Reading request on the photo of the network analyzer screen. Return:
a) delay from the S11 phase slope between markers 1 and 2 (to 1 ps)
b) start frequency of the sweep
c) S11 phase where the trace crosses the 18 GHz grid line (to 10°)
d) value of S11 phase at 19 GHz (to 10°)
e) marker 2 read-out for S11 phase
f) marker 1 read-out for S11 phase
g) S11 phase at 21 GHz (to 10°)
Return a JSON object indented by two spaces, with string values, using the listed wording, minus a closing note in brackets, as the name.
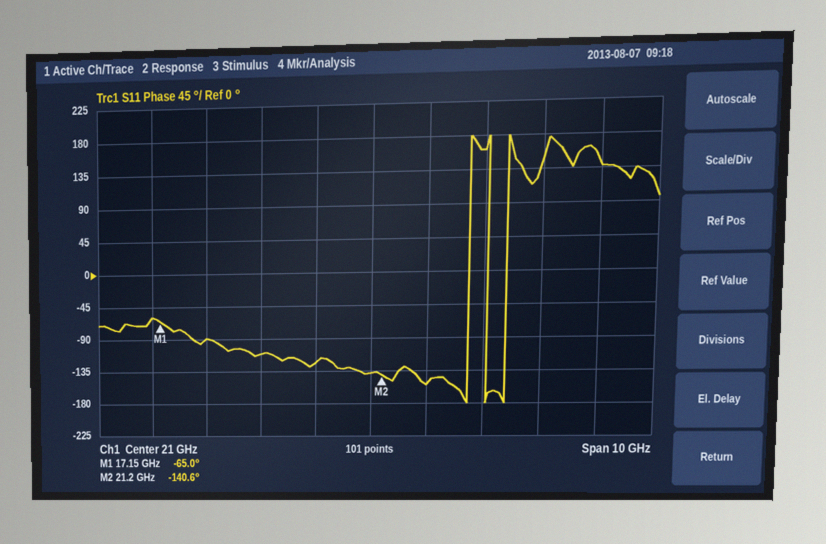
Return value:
{
  "delay from the S11 phase slope between markers 1 and 2": "52 ps",
  "start frequency of the sweep": "16 GHz",
  "S11 phase where the trace crosses the 18 GHz grid line": "-90°",
  "value of S11 phase at 19 GHz": "-110°",
  "marker 2 read-out for S11 phase": "-140.6°",
  "marker 1 read-out for S11 phase": "-65.0°",
  "S11 phase at 21 GHz": "-140°"
}
